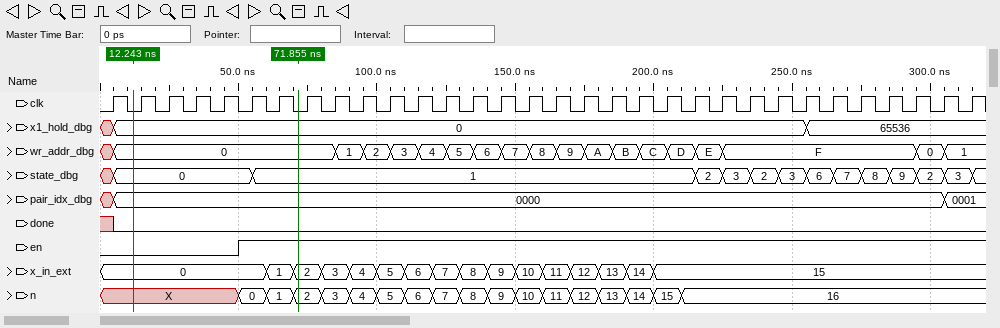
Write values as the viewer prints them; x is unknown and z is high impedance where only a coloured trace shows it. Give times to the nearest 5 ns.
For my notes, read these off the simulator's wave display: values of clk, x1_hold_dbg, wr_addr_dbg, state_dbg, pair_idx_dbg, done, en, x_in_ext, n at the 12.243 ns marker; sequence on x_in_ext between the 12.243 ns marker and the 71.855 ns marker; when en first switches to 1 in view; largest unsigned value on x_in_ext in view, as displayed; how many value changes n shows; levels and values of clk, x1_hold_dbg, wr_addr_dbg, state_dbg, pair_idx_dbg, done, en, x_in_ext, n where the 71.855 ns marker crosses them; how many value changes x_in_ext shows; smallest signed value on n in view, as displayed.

clk=0, x1_hold_dbg=0, wr_addr_dbg=0, state_dbg=0, pair_idx_dbg=0000, done=0, en=0, x_in_ext=0, n=X
0, 1, 2
50 ns
15
17
clk=0, x1_hold_dbg=0, wr_addr_dbg=0, state_dbg=1, pair_idx_dbg=0000, done=0, en=1, x_in_ext=2, n=2
15
0
